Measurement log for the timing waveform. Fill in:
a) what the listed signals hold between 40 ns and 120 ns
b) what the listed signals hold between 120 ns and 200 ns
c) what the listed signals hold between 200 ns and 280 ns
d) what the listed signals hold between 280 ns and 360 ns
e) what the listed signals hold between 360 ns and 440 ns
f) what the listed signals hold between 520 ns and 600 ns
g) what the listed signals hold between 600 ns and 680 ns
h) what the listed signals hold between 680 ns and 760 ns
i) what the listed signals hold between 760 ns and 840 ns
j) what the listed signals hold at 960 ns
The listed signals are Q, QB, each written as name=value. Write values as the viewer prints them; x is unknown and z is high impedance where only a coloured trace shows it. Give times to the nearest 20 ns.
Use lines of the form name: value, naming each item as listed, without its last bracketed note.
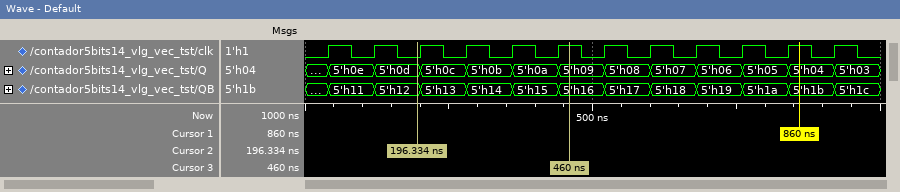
what the listed signals hold between 40 ns and 120 ns: Q=5'h0e, QB=5'h11
what the listed signals hold between 120 ns and 200 ns: Q=5'h0d, QB=5'h12
what the listed signals hold between 200 ns and 280 ns: Q=5'h0c, QB=5'h13
what the listed signals hold between 280 ns and 360 ns: Q=5'h0b, QB=5'h14
what the listed signals hold between 360 ns and 440 ns: Q=5'h0a, QB=5'h15
what the listed signals hold between 520 ns and 600 ns: Q=5'h08, QB=5'h17
what the listed signals hold between 600 ns and 680 ns: Q=5'h07, QB=5'h18
what the listed signals hold between 680 ns and 760 ns: Q=5'h06, QB=5'h19
what the listed signals hold between 760 ns and 840 ns: Q=5'h05, QB=5'h1a
what the listed signals hold at 960 ns: Q=5'h03, QB=5'h1c
